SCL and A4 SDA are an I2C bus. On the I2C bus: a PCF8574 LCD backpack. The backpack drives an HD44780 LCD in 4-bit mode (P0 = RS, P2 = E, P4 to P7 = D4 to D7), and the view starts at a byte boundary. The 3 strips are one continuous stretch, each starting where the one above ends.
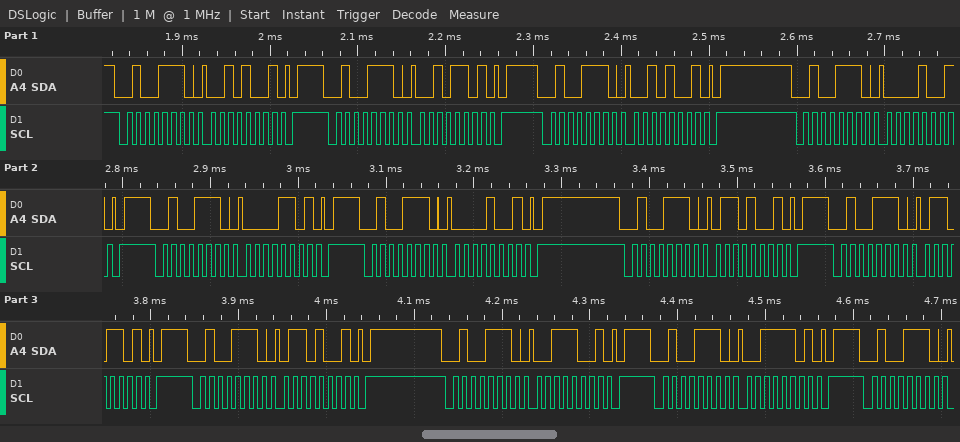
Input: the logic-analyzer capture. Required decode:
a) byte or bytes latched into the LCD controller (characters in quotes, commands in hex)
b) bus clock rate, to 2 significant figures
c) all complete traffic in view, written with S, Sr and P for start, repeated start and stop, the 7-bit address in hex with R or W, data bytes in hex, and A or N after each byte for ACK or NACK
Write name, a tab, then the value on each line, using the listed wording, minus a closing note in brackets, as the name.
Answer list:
byte or bytes latched into the LCD controller	' '
bus clock rate, to 2 significant figures	100 kHz
all complete traffic in view, written with S, Sr and P for start, repeated start and stop, the 7-bit address in hex with R or W, data bytes in hex, and A or N after each byte for ACK or NACK	S 27W A 29 A P S 27W A 2D A P S 27W A 29 A P S 27W A 09 A P S 27W A 0D A P S 27W A 09 A P S 27W A 69 A P S 27W A 6D A P S 27W A 69 A P S 27W A 39 A P S 27W A 3D A P S 27W A
